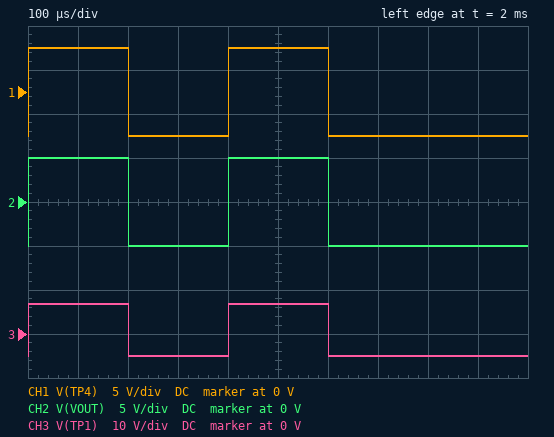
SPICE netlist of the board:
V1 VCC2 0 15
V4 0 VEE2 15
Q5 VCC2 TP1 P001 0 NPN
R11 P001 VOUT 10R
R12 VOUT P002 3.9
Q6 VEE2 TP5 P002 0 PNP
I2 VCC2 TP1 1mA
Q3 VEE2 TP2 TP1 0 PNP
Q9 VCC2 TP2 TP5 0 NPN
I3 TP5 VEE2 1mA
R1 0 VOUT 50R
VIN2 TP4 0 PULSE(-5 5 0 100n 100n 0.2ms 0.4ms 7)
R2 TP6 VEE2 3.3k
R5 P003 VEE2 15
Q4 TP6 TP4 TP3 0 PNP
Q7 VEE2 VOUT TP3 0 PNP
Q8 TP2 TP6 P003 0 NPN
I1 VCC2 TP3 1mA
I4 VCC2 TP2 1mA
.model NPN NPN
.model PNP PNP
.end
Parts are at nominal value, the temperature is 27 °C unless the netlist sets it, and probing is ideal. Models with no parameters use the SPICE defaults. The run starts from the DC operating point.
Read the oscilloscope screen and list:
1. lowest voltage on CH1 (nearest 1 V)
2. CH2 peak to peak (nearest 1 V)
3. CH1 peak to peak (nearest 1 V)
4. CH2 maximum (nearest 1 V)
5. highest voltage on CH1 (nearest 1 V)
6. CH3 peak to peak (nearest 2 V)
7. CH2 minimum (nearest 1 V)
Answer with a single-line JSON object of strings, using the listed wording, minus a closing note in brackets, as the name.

{"lowest voltage on CH1": "-5 V", "CH2 peak to peak": "10 V", "CH1 peak to peak": "10 V", "CH2 maximum": "5 V", "highest voltage on CH1": "5 V", "CH3 peak to peak": "12 V", "CH2 minimum": "-5 V"}
